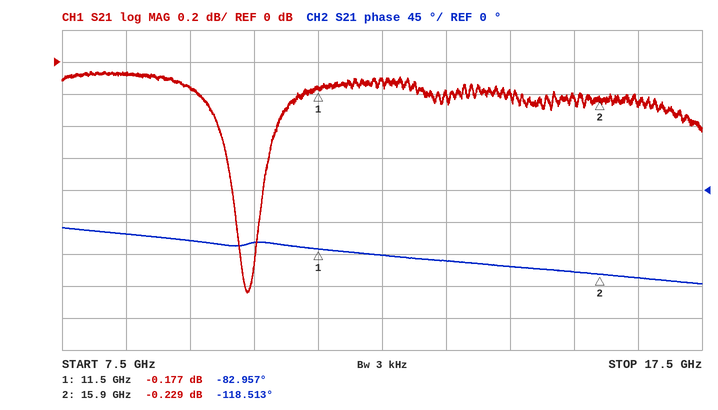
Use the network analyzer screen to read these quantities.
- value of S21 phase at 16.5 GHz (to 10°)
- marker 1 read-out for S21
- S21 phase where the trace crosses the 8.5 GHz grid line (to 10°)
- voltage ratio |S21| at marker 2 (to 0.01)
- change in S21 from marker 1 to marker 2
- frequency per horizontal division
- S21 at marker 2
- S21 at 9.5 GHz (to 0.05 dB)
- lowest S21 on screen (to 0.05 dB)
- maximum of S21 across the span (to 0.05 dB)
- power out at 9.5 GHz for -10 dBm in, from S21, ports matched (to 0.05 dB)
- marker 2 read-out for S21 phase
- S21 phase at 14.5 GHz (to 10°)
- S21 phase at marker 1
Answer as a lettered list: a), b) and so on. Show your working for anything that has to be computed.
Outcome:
a) -120°
b) -0.177 dB
c) -60°
d) 10^(-0.229/20) ≈ 0.97
e) -0.229 − (-0.177) = -0.052 dB
f) 1 GHz
g) -0.229 dB
h) -0.15 dB
i) -1.45 dB
j) -0.05 dB
k) -10 dBm + (-0.15 dB) = -10.15 dBm
l) -118.513°
m) -110°
n) -82.957°
